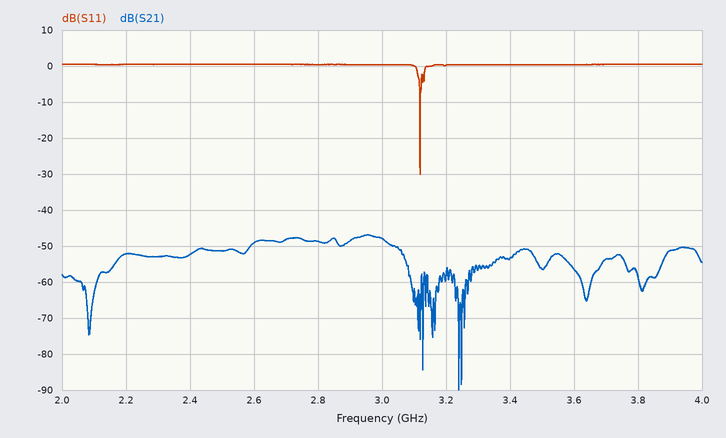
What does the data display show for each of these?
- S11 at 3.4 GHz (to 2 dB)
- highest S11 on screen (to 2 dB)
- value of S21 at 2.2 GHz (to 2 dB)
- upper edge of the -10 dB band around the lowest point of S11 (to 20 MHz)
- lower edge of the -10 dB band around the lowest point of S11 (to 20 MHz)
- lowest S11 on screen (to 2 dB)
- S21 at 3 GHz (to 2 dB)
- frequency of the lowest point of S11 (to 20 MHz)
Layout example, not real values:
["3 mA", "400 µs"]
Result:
["0 dB", "0 dB", "-52 dB", "3.12 GHz", "3.12 GHz", "-30 dB", "-48 dB", "3.12 GHz"]
